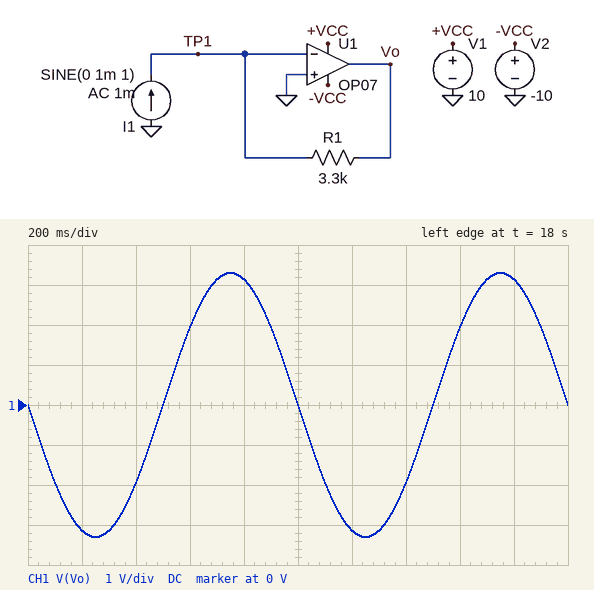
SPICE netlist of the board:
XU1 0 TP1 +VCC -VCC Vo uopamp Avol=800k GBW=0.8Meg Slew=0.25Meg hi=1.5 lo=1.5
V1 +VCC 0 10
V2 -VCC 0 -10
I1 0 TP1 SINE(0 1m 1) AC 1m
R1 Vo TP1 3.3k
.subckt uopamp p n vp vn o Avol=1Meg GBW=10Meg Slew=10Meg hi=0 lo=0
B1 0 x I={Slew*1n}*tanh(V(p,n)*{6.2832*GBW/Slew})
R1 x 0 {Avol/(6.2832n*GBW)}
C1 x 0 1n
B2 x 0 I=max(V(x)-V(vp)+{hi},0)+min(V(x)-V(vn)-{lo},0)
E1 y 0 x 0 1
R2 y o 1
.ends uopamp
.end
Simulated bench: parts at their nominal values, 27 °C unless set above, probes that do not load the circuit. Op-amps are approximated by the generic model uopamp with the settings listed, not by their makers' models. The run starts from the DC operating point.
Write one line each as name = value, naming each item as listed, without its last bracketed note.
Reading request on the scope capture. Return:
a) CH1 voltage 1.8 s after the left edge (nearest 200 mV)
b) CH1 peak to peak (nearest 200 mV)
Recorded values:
CH1 voltage 1.8 s after the left edge = 3.2 V
CH1 peak to peak = 6.6 V
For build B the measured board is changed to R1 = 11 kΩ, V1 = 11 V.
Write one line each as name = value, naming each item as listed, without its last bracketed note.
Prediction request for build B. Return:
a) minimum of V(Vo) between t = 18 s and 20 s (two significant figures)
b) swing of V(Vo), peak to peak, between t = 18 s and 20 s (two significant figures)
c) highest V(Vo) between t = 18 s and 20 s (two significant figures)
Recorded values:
minimum of V(Vo) between t = 18 s and 20 s = -8.5 V
swing of V(Vo), peak to peak, between t = 18 s and 20 s = 18 V
highest V(Vo) between t = 18 s and 20 s = 9.5 V
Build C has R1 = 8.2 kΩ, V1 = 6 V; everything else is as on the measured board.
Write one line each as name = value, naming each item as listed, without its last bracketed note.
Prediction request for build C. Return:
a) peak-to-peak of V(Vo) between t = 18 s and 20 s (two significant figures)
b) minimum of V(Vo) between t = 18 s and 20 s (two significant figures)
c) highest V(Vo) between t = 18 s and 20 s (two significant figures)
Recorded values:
peak-to-peak of V(Vo) between t = 18 s and 20 s = 13 V
minimum of V(Vo) between t = 18 s and 20 s = -8.2 V
highest V(Vo) between t = 18 s and 20 s = 4.5 V
